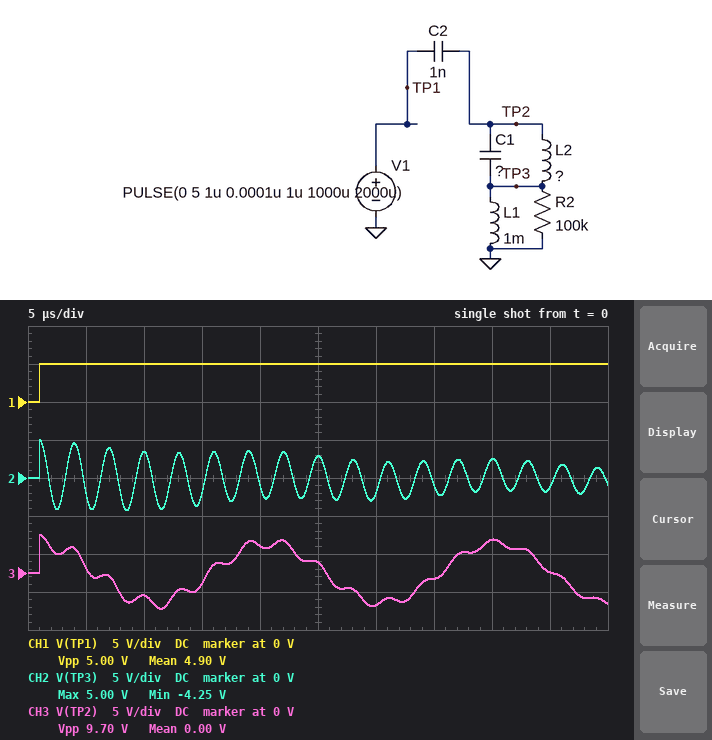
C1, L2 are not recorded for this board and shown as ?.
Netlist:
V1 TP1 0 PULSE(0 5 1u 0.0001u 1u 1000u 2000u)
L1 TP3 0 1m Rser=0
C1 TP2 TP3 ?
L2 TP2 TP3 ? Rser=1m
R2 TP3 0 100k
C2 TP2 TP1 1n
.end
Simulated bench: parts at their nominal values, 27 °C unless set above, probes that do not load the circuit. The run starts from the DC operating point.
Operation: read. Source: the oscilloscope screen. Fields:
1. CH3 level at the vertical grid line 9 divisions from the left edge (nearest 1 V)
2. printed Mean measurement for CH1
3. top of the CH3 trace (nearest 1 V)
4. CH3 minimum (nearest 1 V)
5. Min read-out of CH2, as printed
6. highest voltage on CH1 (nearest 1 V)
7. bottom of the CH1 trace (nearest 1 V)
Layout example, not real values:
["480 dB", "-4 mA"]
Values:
["0 V", "4.90 V", "5 V", "-5 V", "-4.25 V", "5 V", "0 V"]
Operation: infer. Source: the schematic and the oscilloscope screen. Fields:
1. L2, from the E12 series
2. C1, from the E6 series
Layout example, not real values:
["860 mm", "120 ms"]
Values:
["6.8 mH", "330 pF"]
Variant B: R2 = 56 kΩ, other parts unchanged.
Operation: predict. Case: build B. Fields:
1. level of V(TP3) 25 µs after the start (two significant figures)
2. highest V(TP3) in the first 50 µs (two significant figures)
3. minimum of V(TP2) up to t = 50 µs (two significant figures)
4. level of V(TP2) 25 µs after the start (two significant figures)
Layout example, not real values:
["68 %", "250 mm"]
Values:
["2.0 V", "5.0 V", "-4.6 V", "1.2 V"]
